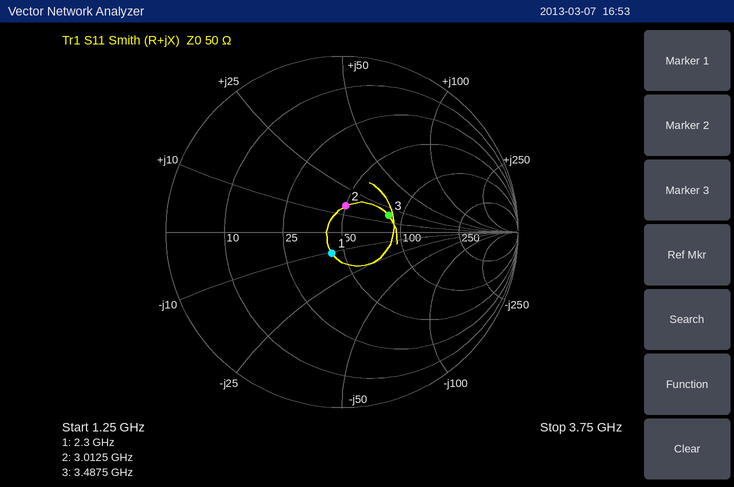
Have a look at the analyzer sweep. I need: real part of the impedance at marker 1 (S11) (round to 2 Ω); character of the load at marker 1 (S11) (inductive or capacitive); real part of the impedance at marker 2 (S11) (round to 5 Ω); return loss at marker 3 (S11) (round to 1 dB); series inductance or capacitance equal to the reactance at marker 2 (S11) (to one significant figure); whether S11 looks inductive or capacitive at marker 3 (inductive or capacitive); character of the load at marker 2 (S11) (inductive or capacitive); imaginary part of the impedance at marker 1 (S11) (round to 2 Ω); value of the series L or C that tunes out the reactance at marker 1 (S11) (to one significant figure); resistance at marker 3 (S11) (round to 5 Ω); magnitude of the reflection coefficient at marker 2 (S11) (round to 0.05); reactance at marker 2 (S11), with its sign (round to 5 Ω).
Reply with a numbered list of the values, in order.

1. 44 Ω
2. capacitive
3. 50 Ω
4. 11 dB
5. 800 pH
6. inductive
7. inductive
8. -10 Ω
9. 700 pH
10. 85 Ω
11. 0.15
12. +15 Ω
